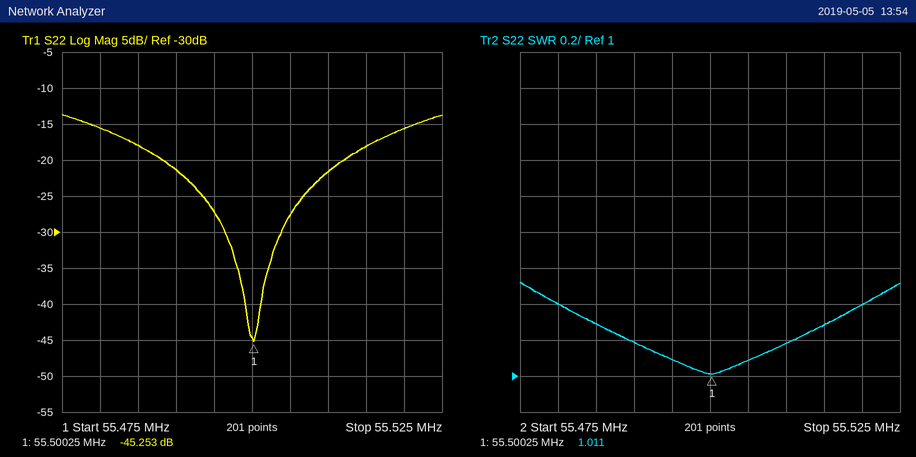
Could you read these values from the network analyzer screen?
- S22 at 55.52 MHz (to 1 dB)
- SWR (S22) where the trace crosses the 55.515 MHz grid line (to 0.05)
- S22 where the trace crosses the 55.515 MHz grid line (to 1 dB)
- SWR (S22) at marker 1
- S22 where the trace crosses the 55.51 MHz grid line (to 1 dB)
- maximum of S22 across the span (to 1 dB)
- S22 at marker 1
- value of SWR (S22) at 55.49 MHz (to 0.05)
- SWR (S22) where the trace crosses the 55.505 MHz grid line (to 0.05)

-16 dB
1.30
-18 dB
1.011
-22 dB
-14 dB
-45.253 dB
1.20
1.10
